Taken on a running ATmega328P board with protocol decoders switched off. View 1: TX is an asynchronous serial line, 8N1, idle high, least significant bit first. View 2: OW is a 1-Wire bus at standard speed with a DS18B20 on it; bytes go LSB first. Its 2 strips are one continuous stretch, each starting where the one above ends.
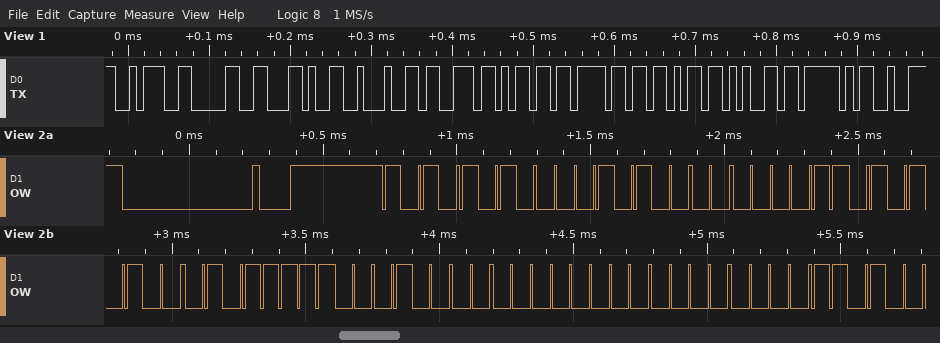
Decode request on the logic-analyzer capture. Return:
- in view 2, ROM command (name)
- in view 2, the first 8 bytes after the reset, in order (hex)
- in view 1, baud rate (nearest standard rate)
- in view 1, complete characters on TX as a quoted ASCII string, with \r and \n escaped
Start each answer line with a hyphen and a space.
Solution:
- Match ROM
- 55 28 C0 2A FA 08 00 00
- 115200 baud
- ":0,\"smoke_"
